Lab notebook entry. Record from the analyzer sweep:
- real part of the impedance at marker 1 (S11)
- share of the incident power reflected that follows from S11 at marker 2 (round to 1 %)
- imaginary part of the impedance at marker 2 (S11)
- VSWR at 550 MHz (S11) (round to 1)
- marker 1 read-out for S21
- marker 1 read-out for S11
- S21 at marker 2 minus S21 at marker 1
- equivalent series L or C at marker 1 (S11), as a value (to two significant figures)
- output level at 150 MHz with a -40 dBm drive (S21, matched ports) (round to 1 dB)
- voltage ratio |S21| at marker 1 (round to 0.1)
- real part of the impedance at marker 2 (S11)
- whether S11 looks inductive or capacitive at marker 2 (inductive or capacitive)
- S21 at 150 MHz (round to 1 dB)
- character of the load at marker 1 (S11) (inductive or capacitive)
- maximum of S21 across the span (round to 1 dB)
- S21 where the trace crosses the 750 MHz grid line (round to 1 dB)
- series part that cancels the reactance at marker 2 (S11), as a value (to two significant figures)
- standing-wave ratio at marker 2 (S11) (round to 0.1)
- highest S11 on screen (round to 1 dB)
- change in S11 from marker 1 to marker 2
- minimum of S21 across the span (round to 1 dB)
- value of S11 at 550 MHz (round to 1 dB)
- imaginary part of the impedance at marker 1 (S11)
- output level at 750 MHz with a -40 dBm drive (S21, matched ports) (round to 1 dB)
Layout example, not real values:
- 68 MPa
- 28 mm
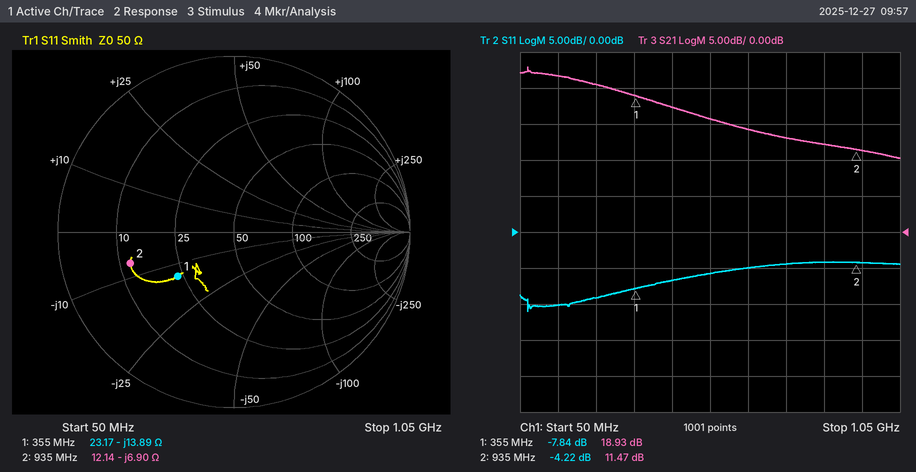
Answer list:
- 23.17 Ω
- 38 %
- -6.90 Ω
- 3
- 18.93 dB
- -7.84 dB
- -7.46 dB
- 32 pF
- -18 dBm
- 8.8
- 12.14 Ω
- capacitive
- 22 dB
- capacitive
- 23 dB
- 13 dB
- 1.2 nH
- 4.2
- -4 dB
- 3.62 dB
- 10 dB
- -6 dB
- -13.89 Ω
- -27 dBm
